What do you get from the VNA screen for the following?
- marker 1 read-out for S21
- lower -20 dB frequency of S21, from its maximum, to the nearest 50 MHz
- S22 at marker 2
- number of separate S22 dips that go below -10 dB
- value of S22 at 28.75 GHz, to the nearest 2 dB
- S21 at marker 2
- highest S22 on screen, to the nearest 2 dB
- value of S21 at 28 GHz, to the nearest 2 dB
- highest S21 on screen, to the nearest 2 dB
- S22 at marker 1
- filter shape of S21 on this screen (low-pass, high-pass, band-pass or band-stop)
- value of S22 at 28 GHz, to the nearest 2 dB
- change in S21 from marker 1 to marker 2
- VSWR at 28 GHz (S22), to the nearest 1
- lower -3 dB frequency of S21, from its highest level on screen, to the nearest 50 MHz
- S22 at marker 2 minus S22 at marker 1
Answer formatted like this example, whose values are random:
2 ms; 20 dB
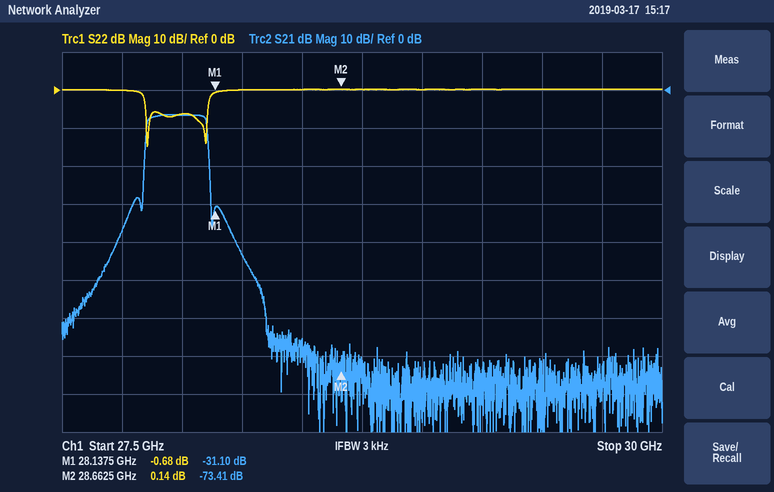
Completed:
-31.10 dB; 27.85 GHz; 0.14 dB; 2; 0 dB; -73.41 dB; 0 dB; -6 dB; -6 dB; -0.68 dB; band-pass; -6 dB; -42.31 dB; 3; 27.85 GHz; 0.82 dB
